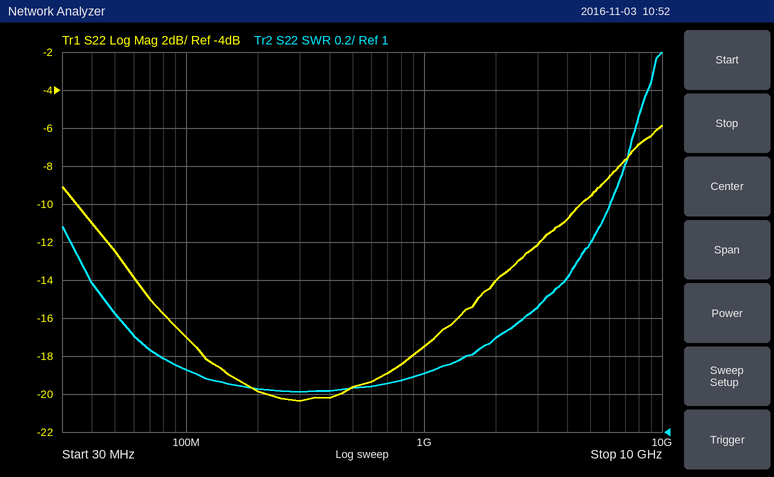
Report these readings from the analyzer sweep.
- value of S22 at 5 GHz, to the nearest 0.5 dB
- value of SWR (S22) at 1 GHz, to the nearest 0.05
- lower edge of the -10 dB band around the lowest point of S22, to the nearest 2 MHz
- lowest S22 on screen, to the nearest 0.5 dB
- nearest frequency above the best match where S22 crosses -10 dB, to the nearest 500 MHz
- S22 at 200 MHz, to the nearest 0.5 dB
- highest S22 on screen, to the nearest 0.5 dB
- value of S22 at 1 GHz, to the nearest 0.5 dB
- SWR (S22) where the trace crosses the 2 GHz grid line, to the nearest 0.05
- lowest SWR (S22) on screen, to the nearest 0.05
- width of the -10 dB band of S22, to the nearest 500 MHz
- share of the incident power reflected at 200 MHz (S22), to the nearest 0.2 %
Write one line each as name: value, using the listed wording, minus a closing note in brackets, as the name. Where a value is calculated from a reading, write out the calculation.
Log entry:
value of S22 at 5 GHz, to the nearest 0.5 dB: -9.5 dB
value of SWR (S22) at 1 GHz, to the nearest 0.05: 1.30
lower edge of the -10 dB band around the lowest point of S22, to the nearest 2 MHz: 34 MHz
lowest S22 on screen, to the nearest 0.5 dB: -20.5 dB
nearest frequency above the best match where S22 crosses -10 dB, to the nearest 500 MHz: 4.5 GHz
S22 at 200 MHz, to the nearest 0.5 dB: -20.0 dB
highest S22 on screen, to the nearest 0.5 dB: -6.0 dB
value of S22 at 1 GHz, to the nearest 0.5 dB: -17.5 dB
SWR (S22) where the trace crosses the 2 GHz grid line, to the nearest 0.05: 1.50
lowest SWR (S22) on screen, to the nearest 0.05: 1.20
width of the -10 dB band of S22, to the nearest 500 MHz: 4.5 GHz − 34 MHz = 4.466 GHz
share of the incident power reflected at 200 MHz (S22), to the nearest 0.2 %: 10^(-20/10) ≈ 1.0 %
